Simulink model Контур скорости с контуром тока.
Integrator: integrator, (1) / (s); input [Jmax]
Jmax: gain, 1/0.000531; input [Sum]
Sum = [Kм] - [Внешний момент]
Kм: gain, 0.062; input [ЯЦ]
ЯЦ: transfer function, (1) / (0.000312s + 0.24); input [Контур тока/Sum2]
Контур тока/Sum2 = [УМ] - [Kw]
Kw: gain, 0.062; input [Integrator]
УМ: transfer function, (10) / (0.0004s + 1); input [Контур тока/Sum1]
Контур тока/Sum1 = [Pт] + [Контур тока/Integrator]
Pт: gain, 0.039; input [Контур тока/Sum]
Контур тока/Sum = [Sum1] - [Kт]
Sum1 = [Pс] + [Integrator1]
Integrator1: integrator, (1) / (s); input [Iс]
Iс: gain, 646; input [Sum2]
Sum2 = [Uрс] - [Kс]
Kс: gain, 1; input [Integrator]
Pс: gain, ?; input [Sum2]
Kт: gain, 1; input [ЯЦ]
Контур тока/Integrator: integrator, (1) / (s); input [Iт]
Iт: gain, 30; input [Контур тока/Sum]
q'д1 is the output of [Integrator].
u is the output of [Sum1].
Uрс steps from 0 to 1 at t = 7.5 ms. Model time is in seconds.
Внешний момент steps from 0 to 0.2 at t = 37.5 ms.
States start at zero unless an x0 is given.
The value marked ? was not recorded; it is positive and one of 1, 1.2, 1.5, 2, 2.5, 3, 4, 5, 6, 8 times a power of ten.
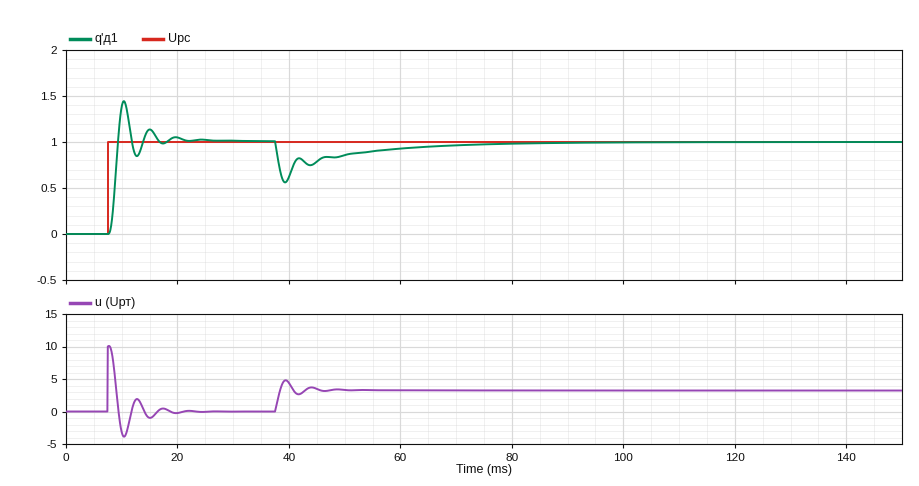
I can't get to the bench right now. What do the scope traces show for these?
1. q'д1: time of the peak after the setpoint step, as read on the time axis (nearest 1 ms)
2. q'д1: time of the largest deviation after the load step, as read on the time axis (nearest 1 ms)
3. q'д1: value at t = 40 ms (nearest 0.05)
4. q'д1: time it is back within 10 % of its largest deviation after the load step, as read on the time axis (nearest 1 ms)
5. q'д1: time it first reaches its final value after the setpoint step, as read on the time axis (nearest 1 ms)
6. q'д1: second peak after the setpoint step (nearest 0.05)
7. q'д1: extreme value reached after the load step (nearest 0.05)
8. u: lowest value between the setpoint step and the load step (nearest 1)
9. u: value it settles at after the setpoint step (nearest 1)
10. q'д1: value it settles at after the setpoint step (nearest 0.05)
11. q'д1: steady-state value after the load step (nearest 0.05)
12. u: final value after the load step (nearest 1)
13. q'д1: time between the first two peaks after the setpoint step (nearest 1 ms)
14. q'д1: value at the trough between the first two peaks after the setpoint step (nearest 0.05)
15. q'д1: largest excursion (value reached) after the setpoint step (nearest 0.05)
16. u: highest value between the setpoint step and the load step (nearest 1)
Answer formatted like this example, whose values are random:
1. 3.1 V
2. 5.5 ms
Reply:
1. 10 ms
2. 39 ms
3. 0.60
4. 67 ms
5. 9 ms
6. 1.15
7. 0.55
8. -4
9. 0
10. 1.00
11. 1.00
12. 3
13. 5 ms
14. 0.85
15. 1.45
16. 10
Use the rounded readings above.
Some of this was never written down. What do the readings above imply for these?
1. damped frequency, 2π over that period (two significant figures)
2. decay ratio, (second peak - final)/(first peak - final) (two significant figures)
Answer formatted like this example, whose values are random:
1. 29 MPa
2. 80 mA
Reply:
1. 1.3 rad/ms
2. 0.33
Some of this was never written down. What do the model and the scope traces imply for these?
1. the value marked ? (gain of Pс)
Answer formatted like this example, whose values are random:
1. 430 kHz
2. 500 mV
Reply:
1. 10
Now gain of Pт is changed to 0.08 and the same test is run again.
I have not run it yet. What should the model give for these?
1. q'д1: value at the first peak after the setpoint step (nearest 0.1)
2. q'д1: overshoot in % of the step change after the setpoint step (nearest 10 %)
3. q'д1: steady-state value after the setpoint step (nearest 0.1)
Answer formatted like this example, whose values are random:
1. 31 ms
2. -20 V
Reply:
1. 1.2
2. 20 %
3. 1.0
